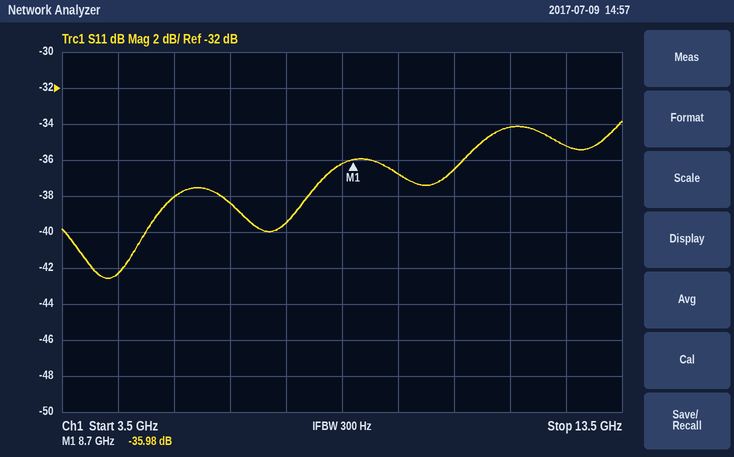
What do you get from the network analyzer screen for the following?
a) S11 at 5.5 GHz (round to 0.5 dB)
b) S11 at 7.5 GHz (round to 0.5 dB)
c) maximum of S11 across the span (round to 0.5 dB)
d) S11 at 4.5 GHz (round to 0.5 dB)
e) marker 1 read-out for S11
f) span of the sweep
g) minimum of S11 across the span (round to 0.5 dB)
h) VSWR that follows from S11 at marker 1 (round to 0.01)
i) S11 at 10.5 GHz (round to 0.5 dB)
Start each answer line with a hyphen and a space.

- -38.0 dB
- -39.5 dB
- -34.0 dB
- -42.5 dB
- -35.98 dB
- 10 GHz
- -42.5 dB
- 1.03
- -36.5 dB
